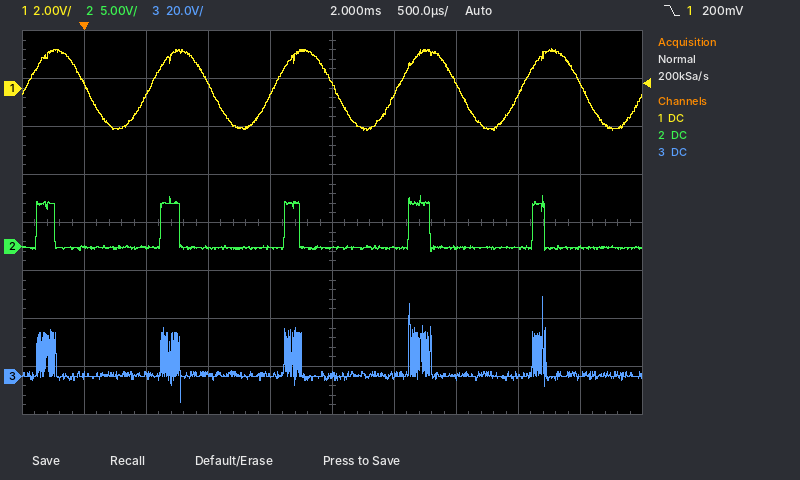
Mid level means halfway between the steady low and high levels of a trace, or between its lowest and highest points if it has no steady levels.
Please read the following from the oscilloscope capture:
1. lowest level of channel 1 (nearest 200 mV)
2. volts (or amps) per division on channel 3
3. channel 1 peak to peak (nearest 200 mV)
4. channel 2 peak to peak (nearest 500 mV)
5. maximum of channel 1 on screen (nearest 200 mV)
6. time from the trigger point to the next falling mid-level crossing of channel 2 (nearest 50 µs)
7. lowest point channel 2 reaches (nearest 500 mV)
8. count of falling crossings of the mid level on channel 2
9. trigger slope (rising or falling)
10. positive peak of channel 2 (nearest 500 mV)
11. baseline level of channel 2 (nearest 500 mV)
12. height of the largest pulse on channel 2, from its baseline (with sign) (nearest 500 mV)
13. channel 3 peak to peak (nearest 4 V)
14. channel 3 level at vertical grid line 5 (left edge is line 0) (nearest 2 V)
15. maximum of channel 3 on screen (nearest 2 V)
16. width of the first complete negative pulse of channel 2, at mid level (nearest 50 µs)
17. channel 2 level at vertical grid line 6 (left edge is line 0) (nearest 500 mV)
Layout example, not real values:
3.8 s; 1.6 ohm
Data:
-1.8 V; 20 V; 3.4 V; 6.0 V; 1.6 V; 750 µs; -500 mV; 5; falling; 5.5 V; 0.0 V; +5.5 V; 44 V; 0 V; 34 V; 850 µs; 0.0 V
